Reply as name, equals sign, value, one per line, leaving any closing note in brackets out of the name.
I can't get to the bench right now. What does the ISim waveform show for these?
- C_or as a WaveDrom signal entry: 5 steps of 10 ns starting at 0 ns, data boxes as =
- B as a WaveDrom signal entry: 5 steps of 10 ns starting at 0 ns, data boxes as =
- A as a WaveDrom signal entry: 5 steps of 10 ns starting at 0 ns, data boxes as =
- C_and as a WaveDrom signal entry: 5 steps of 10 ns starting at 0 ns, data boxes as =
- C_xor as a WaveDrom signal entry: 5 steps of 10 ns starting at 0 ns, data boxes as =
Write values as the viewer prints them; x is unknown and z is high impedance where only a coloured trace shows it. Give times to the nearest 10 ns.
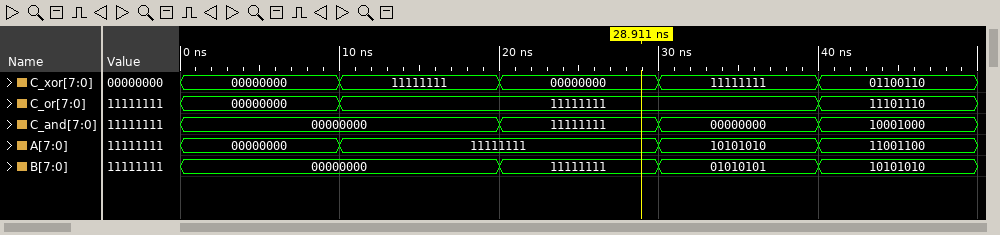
C_or as a WaveDrom signal entry: 5 steps of 10 ns starting at 0 ns, data boxes as = = {name: 'C_or', wave: '==..=', data: '00000000 11111111 11101110'}
B as a WaveDrom signal entry: 5 steps of 10 ns starting at 0 ns, data boxes as = = {name: 'B', wave: '=.===', data: '00000000 11111111 01010101 10101010'}
A as a WaveDrom signal entry: 5 steps of 10 ns starting at 0 ns, data boxes as = = {name: 'A', wave: '==.==', data: '00000000 11111111 10101010 11001100'}
C_and as a WaveDrom signal entry: 5 steps of 10 ns starting at 0 ns, data boxes as = = {name: 'C_and', wave: '=.===', data: '00000000 11111111 00000000 10001000'}
C_xor as a WaveDrom signal entry: 5 steps of 10 ns starting at 0 ns, data boxes as = = {name: 'C_xor', wave: '=====', data: '00000000 11111111 00000000 11111111 01100110'}
